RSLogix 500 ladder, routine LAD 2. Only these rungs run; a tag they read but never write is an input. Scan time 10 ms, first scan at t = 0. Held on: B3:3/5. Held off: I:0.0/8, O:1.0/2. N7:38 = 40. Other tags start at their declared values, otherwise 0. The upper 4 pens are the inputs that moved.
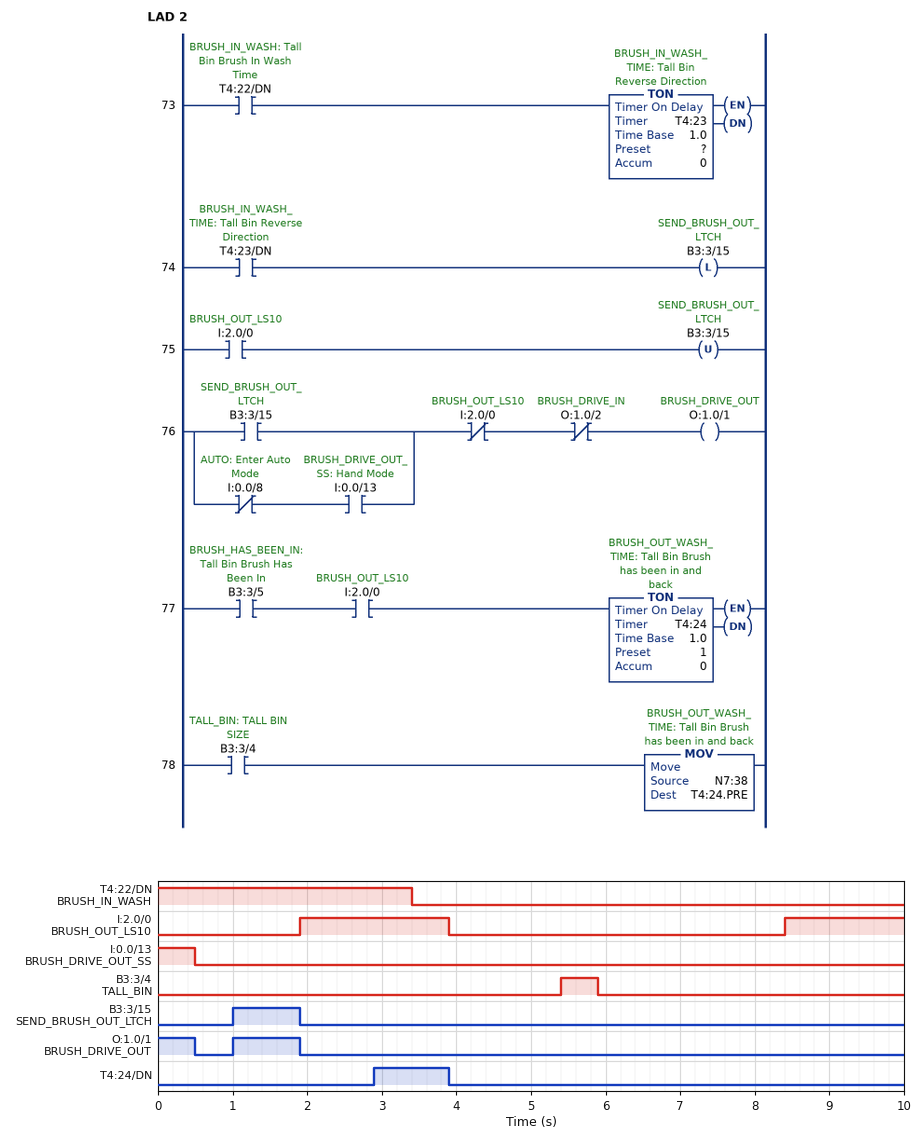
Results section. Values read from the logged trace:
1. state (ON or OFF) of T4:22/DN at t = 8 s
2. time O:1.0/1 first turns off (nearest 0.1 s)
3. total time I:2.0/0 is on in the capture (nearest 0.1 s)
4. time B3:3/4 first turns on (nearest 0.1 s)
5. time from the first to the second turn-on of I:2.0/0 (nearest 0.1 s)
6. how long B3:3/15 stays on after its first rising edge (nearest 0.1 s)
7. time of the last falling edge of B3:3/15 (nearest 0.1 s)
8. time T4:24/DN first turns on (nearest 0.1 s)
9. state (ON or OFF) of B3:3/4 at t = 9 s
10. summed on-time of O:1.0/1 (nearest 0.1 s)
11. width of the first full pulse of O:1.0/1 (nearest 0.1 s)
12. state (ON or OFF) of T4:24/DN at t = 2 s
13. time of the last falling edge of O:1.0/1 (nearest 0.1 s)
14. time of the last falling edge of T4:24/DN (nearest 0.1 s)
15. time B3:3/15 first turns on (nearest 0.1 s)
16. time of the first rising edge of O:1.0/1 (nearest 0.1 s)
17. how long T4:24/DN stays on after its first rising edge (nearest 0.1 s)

OFF
0.5 s
3.6 s
5.4 s
6.5 s
0.9 s
1.9 s
2.9 s
OFF
1.4 s
0.9 s
OFF
1.9 s
3.9 s
1.0 s
1.0 s
1.0 s
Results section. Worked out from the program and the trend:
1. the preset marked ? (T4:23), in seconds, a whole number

1 s
